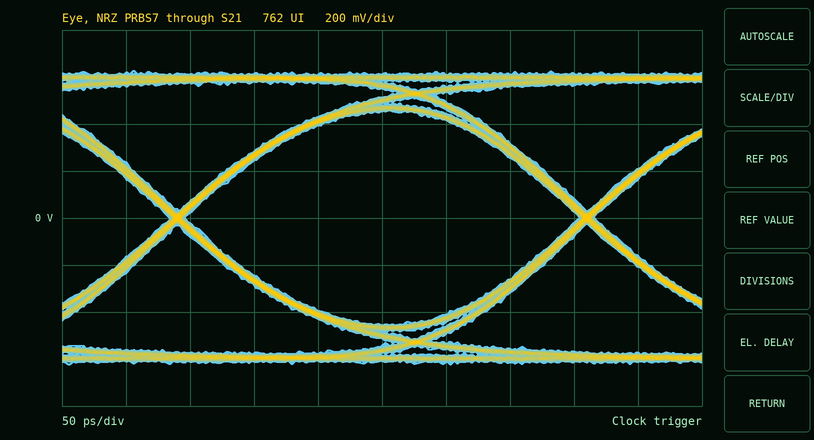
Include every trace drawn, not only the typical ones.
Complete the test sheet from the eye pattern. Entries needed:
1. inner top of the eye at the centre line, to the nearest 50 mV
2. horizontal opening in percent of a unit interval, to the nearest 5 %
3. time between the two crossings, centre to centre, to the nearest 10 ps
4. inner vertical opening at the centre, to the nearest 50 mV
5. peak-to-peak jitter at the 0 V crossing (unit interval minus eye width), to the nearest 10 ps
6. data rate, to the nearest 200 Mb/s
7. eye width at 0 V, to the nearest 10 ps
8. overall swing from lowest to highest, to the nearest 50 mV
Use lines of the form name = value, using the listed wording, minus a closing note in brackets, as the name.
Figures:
inner top of the eye at the centre line, to the nearest 50 mV = 450 mV
horizontal opening in percent of a unit interval, to the nearest 5 % = 95 %
time between the two crossings, centre to centre, to the nearest 10 ps = 320 ps
inner vertical opening at the centre, to the nearest 50 mV = 900 mV
peak-to-peak jitter at the 0 V crossing (unit interval minus eye width), to the nearest 10 ps = 10 ps
data rate, to the nearest 200 Mb/s = 3.2 Gb/s
eye width at 0 V, to the nearest 10 ps = 310 ps
overall swing from lowest to highest, to the nearest 50 mV = 1.25 V
